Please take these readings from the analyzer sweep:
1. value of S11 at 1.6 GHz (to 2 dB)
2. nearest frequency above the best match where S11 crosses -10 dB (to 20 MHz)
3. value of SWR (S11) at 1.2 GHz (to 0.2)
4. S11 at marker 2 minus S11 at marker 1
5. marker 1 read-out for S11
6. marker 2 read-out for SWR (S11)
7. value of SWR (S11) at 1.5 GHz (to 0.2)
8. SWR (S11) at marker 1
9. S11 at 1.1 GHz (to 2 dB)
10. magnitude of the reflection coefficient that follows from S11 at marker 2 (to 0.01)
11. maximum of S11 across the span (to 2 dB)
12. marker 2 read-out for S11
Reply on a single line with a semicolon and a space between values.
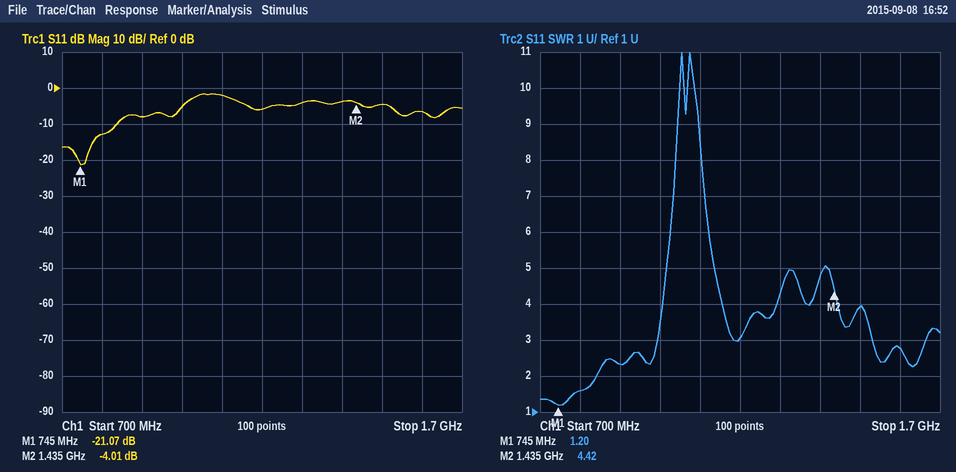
-6 dB; 840 MHz; 3.0; 17.06 dB; -21.07 dB; 4.42; 4.0; 1.20; -2 dB; 0.63; -2 dB; -4.01 dB
